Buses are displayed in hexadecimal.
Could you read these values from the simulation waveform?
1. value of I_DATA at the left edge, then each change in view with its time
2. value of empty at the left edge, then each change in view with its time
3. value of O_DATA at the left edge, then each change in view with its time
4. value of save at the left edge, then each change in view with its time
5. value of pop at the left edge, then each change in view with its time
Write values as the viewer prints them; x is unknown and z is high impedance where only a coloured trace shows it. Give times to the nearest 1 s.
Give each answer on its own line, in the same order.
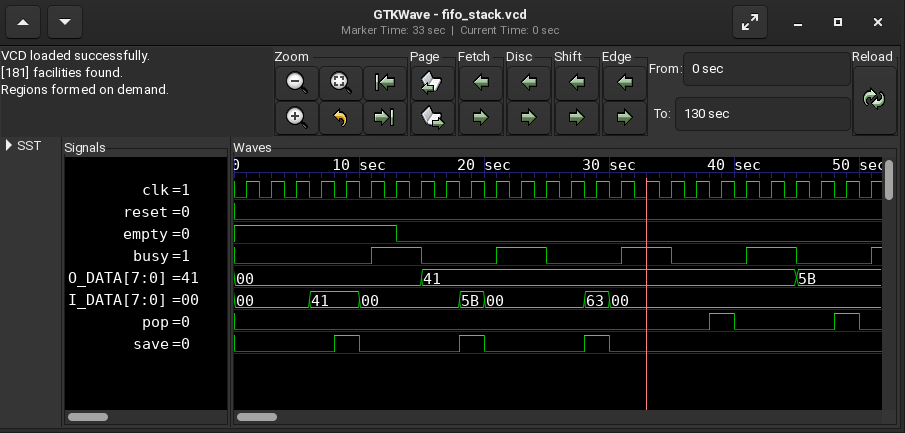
00, 41 at 6 s, 00 at 10 s, 5B at 18 s, 00 at 20 s, 63 at 28 s, 00 at 30 s
1, 0 at 13 s
00, 41 at 15 s, 5B at 45 s
0, 1 at 8 s, 0 at 10 s, 1 at 18 s, 0 at 20 s, 1 at 28 s, 0 at 30 s
0, 1 at 38 s, 0 at 40 s, 1 at 48 s, 0 at 50 s
